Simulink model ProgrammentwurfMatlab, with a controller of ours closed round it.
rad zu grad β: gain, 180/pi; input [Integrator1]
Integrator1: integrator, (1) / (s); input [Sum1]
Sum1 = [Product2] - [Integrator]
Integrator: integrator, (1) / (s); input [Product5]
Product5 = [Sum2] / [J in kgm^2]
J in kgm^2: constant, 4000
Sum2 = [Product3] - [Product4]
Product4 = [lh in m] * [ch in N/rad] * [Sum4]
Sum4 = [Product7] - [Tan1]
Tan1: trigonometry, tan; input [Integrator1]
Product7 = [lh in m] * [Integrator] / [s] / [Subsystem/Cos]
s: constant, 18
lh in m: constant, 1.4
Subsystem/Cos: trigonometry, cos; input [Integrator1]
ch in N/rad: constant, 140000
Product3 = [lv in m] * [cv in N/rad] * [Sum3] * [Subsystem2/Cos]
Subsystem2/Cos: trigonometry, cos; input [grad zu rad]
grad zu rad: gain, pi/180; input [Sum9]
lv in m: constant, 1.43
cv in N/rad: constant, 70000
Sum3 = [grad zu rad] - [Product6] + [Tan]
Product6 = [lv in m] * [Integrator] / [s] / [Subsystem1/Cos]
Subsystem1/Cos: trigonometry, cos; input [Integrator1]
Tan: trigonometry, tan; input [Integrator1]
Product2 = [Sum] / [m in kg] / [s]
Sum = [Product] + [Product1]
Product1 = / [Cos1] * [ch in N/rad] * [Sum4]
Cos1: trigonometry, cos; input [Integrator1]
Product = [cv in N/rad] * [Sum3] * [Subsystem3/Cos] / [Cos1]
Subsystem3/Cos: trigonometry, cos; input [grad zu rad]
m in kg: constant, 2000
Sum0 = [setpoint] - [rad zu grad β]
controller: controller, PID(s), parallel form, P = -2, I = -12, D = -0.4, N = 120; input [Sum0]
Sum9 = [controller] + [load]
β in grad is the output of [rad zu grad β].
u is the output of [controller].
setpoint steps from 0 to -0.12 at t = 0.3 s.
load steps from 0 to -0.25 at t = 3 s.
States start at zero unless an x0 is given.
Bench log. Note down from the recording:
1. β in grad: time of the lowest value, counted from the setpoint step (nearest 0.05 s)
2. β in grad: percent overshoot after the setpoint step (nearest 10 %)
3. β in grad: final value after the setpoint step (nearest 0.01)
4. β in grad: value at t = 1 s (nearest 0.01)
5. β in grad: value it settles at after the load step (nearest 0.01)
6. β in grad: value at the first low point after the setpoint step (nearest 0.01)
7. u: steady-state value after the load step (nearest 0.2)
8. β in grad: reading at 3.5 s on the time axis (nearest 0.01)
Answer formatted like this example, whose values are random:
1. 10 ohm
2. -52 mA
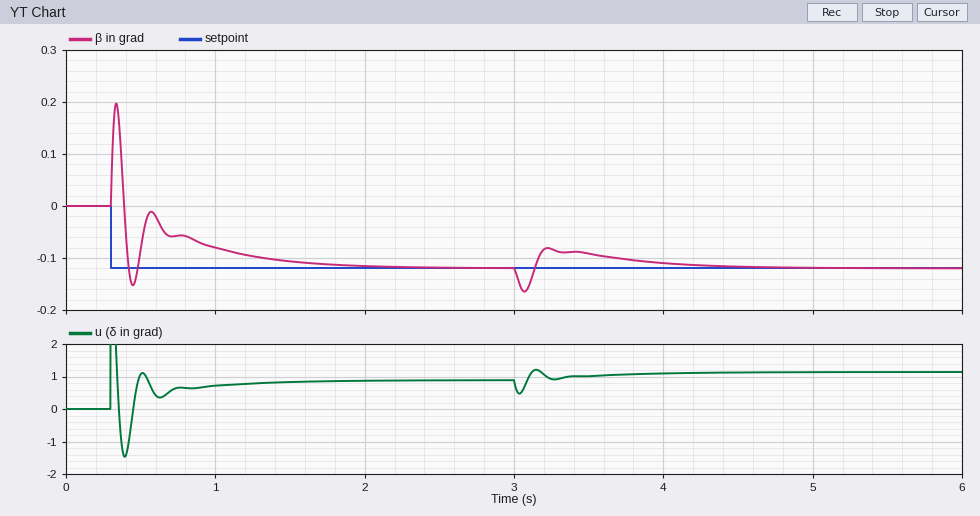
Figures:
1. 0.15 s
2. 30 %
3. -0.12
4. -0.08
5. -0.12
6. -0.15
7. 1.2
8. -0.09
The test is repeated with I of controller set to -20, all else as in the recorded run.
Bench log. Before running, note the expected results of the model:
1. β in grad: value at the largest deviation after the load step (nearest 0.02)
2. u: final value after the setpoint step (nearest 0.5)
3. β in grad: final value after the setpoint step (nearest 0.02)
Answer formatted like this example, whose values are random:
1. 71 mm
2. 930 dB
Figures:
1. -0.16
2. 1.0
3. -0.12
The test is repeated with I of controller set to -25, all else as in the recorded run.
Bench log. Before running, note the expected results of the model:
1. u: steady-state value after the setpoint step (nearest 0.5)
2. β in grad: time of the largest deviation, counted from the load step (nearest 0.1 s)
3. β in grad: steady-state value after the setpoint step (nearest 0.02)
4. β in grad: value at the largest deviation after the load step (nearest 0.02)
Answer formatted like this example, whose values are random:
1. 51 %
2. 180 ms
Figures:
1. 1.0
2. 0.3 s
3. -0.12
4. -0.08
